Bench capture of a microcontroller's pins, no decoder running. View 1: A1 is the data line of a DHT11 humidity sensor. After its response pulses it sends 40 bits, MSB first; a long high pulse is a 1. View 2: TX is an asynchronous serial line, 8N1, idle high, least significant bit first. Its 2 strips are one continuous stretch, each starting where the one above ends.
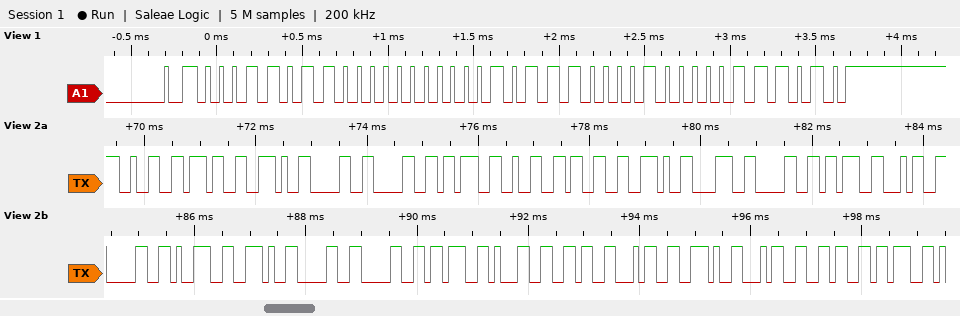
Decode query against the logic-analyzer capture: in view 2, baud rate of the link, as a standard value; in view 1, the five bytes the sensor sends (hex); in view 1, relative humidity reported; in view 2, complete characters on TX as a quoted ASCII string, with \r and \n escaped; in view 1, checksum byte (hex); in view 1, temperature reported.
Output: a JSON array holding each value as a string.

["9600 baud", "1B 00 17 08 3A", "27 %", "\"27.00;23.80;409.00;164.46;\"", "0x3A", "23.8 °C"]
